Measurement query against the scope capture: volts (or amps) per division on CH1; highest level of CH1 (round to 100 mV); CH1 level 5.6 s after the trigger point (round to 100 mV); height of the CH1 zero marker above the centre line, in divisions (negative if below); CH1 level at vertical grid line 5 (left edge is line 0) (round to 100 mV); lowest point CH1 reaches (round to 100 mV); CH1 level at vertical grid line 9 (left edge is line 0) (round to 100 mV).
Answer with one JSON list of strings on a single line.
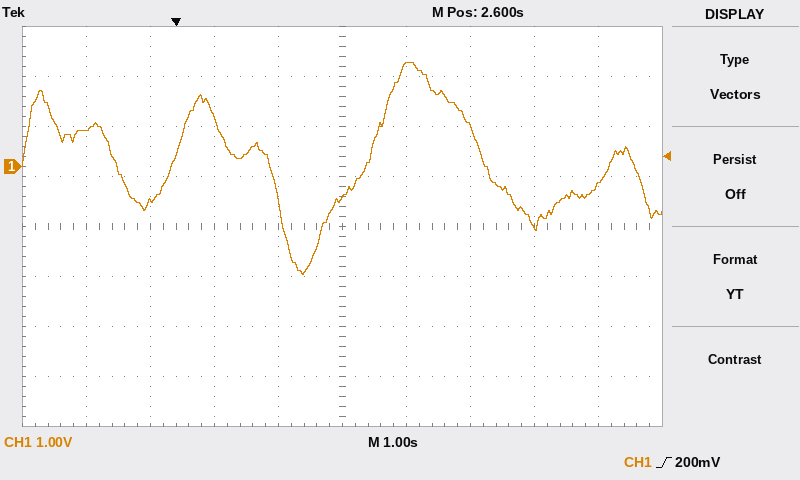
["1 V", "2.1 V", "-1.2 V", "+1.2 div", "-600 mV", "-2.2 V", "-400 mV"]
